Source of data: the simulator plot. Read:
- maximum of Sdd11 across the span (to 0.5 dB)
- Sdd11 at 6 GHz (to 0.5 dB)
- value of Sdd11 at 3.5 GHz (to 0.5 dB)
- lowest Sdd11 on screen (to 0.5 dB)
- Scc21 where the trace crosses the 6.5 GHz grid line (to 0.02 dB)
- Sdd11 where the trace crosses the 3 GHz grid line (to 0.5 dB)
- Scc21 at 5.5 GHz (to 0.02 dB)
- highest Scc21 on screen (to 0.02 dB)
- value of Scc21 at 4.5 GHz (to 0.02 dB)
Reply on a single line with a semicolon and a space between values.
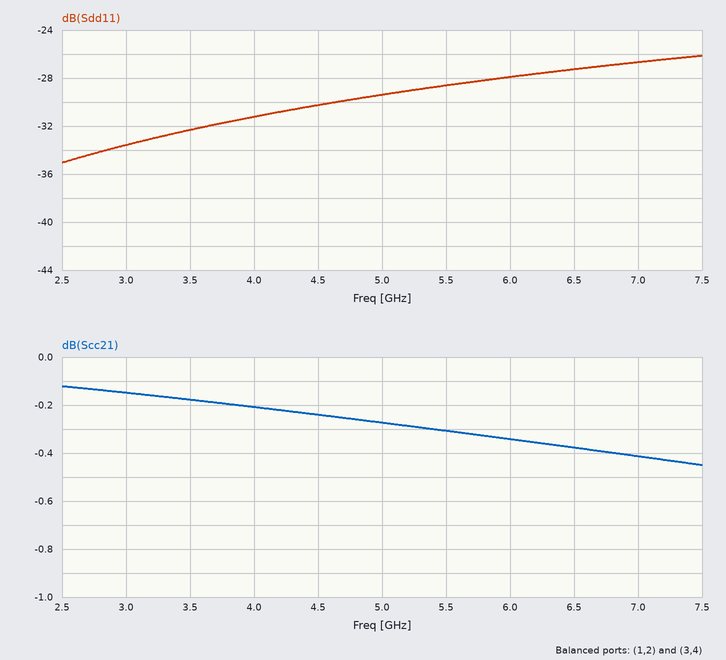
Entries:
-26.0 dB; -28.0 dB; -32.5 dB; -35.0 dB; -0.38 dB; -33.5 dB; -0.30 dB; -0.12 dB; -0.24 dB
